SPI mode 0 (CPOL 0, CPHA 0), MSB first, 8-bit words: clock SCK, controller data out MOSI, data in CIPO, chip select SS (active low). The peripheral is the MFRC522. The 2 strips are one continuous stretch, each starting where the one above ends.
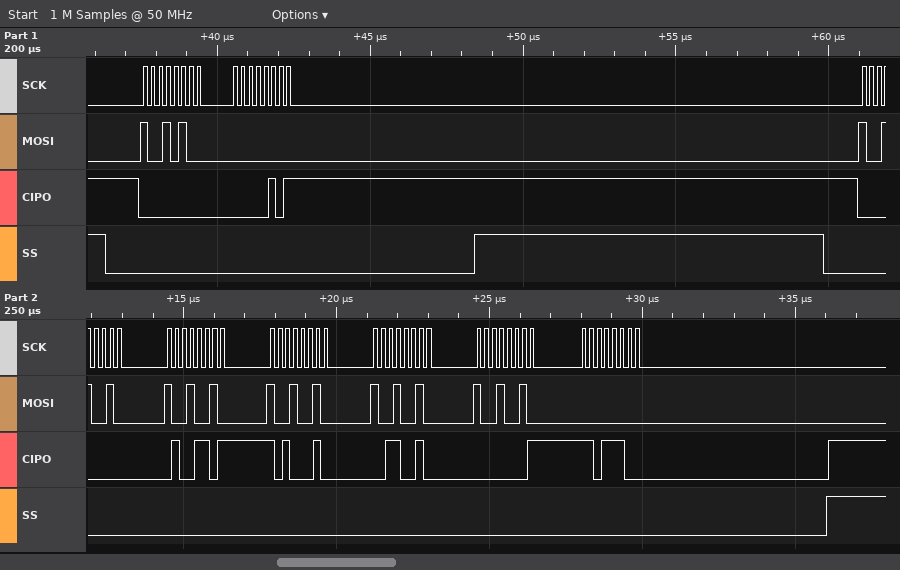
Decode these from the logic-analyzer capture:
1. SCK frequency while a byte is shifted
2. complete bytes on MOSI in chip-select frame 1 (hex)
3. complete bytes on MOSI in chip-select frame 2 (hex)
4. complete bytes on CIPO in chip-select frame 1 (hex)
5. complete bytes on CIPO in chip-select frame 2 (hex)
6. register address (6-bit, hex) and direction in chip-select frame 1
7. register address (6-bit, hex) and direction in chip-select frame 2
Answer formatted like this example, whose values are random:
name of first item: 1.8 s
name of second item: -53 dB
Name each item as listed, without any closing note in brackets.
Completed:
SCK frequency while a byte is shifted: 4 MHz
complete bytes on MOSI in chip-select frame 1: 94 00
complete bytes on MOSI in chip-select frame 2: 92 92 92 92 92 00
complete bytes on CIPO in chip-select frame 1: 00 05
complete bytes on CIPO in chip-select frame 2: 00 4D A2 32 01 DC
register address (6-bit, hex) and direction in chip-select frame 1: 0x0A read
register address (6-bit, hex) and direction in chip-select frame 2: 0x09 read
